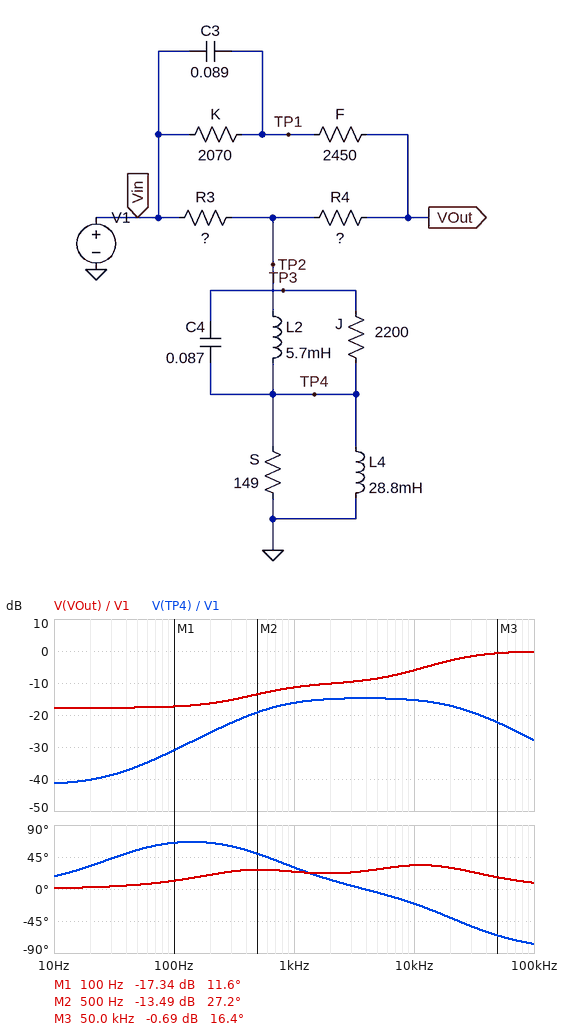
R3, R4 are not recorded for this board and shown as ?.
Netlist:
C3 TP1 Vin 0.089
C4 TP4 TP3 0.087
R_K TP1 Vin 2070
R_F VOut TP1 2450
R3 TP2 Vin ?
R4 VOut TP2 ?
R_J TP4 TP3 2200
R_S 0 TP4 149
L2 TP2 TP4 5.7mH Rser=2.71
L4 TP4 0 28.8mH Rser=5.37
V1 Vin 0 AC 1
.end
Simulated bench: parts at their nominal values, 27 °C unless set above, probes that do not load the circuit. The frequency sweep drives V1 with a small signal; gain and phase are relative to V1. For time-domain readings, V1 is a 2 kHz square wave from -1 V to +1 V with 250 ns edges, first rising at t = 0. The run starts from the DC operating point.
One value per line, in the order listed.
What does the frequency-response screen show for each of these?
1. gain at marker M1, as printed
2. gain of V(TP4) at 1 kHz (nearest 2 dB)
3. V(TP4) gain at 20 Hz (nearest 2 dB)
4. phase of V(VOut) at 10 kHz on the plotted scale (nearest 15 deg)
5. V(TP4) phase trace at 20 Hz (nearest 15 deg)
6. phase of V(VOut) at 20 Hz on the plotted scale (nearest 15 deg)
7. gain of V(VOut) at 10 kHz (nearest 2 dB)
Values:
-17.34 dB
-16 dB
-40 dB
30 deg
30 deg
0 deg
-6 dB
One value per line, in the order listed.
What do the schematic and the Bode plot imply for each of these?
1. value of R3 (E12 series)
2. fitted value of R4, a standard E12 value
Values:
820 Ω
330 Ω
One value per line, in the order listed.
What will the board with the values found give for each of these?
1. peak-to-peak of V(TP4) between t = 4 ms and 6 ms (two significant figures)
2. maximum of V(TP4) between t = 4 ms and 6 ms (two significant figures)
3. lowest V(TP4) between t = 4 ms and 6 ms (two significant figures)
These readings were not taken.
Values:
490 mV
250 mV
-250 mV
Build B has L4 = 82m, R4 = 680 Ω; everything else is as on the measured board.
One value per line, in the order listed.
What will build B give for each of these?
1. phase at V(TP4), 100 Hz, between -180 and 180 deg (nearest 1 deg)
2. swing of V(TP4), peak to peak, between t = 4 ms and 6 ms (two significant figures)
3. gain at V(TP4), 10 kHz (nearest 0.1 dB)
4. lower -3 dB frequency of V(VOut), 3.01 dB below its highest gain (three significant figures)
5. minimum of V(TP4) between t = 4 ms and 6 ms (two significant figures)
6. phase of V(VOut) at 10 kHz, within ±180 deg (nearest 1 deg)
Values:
62 deg
420 mV
-15.4 dB
19.1 kHz
-210 mV
27 deg
